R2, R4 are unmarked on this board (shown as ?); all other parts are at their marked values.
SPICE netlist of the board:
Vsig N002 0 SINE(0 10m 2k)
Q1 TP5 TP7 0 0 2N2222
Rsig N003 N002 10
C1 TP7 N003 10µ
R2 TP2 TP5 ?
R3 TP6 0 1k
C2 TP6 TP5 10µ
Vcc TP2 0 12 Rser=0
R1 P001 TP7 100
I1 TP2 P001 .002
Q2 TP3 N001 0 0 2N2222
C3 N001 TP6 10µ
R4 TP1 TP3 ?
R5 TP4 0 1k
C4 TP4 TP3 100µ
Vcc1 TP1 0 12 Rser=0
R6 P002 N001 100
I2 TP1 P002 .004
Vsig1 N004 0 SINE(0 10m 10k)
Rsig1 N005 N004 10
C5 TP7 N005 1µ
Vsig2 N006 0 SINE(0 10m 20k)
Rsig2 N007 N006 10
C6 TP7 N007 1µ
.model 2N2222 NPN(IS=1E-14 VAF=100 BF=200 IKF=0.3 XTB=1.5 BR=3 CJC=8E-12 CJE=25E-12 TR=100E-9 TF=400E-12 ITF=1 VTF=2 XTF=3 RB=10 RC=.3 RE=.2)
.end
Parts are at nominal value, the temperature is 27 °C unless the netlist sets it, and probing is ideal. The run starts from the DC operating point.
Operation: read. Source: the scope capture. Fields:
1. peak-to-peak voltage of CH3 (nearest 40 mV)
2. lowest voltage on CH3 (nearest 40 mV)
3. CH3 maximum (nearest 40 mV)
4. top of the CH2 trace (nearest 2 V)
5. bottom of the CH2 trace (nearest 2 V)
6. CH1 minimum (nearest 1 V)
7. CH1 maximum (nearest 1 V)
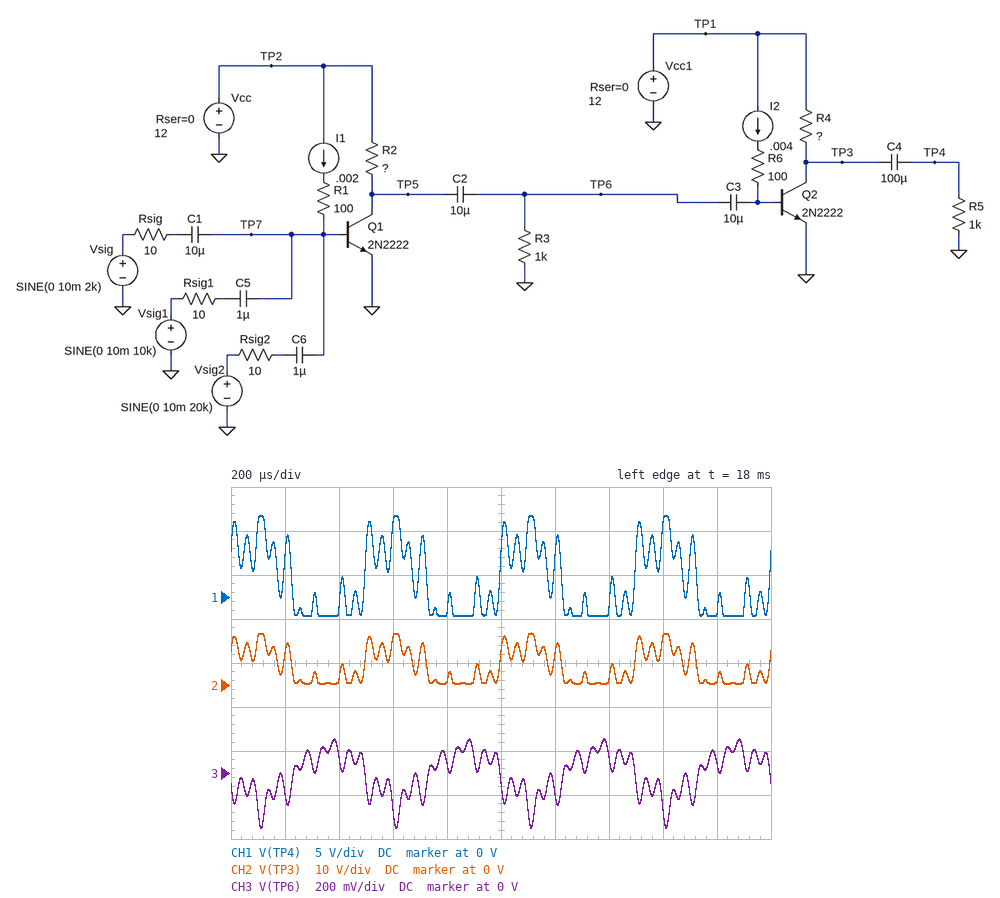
400 mV
-240 mV
160 mV
12 V
0 V
-2 V
9 V
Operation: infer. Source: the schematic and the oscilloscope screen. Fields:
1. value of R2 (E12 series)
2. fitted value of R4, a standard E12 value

12 Ω
27 Ω
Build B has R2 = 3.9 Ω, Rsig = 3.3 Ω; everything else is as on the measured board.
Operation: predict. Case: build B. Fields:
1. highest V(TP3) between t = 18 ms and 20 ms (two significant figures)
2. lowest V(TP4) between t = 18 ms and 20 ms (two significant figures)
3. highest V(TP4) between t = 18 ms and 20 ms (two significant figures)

6.0 V
-1.8 V
3.8 V
